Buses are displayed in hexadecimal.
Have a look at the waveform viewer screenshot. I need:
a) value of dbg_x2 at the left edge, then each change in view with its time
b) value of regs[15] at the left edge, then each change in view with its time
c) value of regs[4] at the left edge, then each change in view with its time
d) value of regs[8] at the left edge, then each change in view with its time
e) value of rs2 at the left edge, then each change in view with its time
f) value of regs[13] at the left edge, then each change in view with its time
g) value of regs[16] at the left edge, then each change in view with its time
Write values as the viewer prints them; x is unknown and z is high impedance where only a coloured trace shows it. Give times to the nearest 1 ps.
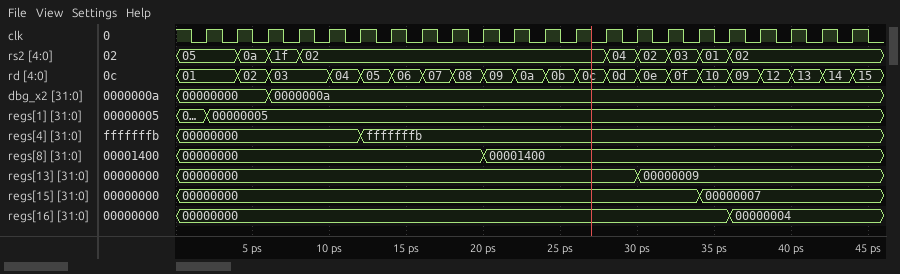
00000000, 0000000a at 6 ps
00000000, 00000007 at 34 ps
00000000, fffffffb at 12 ps
00000000, 00001400 at 20 ps
05, 0a at 4 ps, 1f at 6 ps, 02 at 8 ps, 04 at 28 ps, 02 at 30 ps, 03 at 32 ps, 01 at 34 ps, 02 at 36 ps
00000000, 00000009 at 30 ps
00000000, 00000004 at 36 ps
